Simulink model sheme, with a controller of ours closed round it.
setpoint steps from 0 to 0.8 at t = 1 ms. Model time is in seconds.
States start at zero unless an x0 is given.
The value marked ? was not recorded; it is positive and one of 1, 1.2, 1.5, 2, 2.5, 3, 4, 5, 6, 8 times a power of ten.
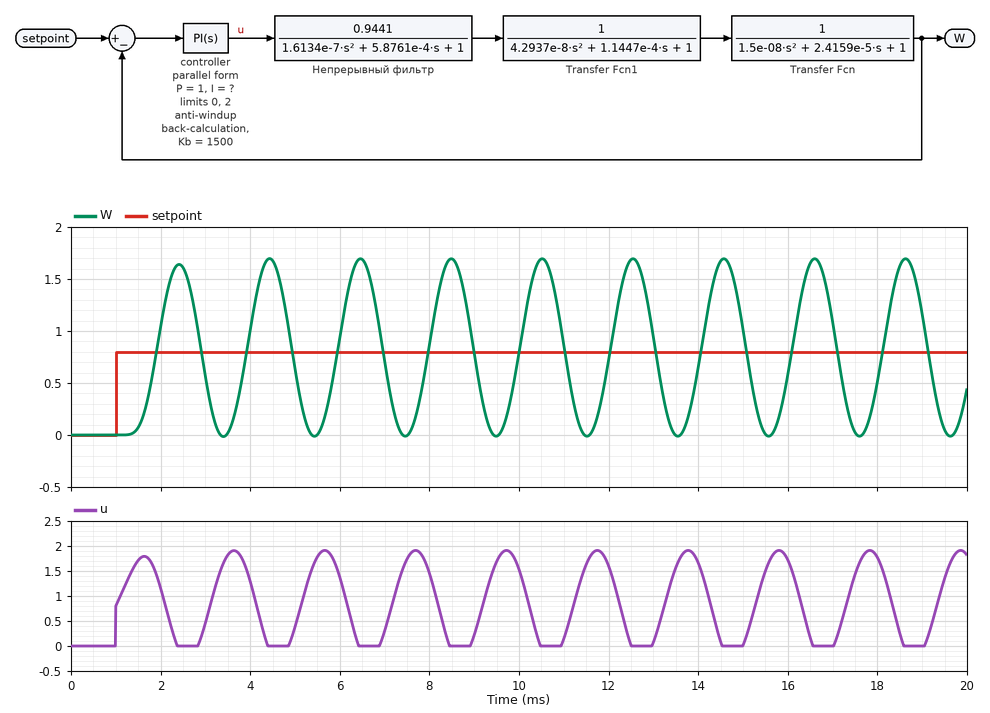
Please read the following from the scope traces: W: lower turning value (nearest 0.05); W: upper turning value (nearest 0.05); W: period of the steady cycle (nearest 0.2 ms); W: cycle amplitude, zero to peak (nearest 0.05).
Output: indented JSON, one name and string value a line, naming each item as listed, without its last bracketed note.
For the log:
{
  "W: lower turning value": "0.00",
  "W: upper turning value": "1.70",
  "W: period of the steady cycle": "2.0 ms",
  "W: cycle amplitude, zero to peak": "0.85"
}
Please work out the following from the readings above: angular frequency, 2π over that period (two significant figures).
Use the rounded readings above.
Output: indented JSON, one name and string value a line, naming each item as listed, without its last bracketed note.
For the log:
{
  "angular frequency, 2π over that period": "3.1 rad/ms"
}
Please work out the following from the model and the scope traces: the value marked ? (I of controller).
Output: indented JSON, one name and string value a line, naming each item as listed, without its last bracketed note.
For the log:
{
  "the value marked ?": "2500"
}
